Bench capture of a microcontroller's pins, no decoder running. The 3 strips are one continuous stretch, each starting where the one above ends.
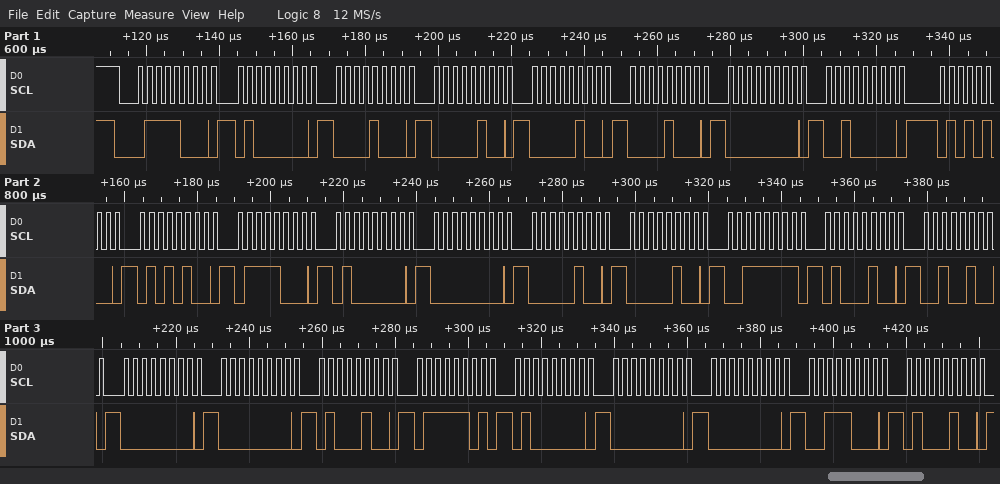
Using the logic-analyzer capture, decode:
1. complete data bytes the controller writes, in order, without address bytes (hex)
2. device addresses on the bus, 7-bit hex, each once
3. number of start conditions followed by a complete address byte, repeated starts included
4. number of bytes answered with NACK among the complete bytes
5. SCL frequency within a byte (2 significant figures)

40 08 04 04 08 00 20 54 54 78 40 00 04 04 3F 44 24 00 00 44 7D 40 00 00 38 44
0x3C
1
0
400 kHz
